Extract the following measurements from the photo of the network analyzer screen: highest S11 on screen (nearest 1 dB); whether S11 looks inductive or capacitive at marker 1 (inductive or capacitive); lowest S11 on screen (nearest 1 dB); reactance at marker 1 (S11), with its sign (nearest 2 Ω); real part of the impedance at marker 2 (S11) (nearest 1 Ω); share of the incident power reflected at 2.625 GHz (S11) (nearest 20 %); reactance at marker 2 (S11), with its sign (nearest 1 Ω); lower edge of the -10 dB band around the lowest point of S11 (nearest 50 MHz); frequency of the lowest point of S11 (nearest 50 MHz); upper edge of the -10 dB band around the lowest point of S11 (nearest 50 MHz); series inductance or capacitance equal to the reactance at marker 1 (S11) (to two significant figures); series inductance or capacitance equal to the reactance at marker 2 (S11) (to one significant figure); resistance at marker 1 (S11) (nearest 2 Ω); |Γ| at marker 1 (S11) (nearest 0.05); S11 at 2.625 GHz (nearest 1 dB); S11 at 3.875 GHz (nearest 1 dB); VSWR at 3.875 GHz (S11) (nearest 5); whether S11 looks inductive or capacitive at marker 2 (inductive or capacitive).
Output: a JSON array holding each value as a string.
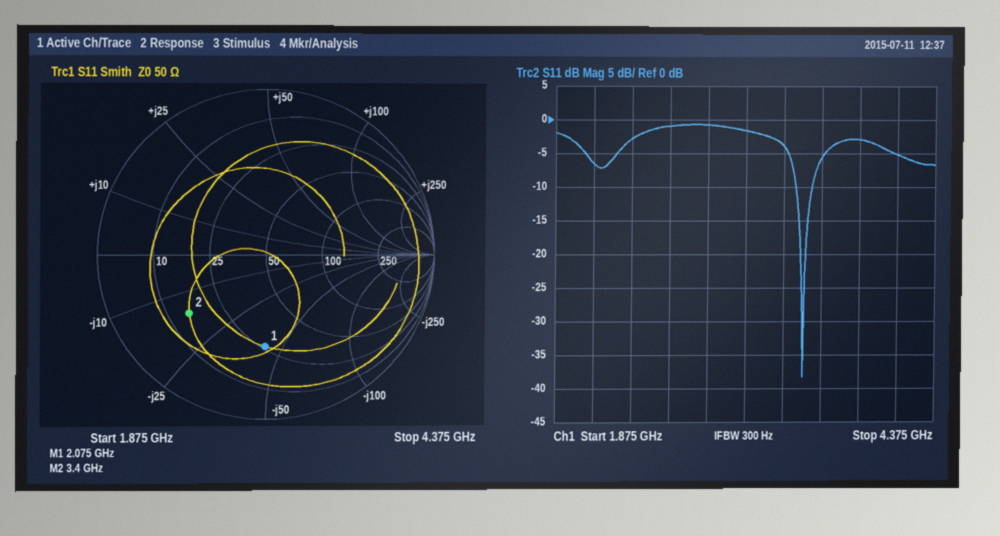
["-1 dB", "capacitive", "-38 dB", "-42 Ω", "15 Ω", "80 %", "-16 Ω", "3.45 GHz", "3.50 GHz", "3.55 GHz", "1.8 pF", "3 pF", "26 Ω", "0.55", "-1 dB", "-3 dB", "5", "capacitive"]
